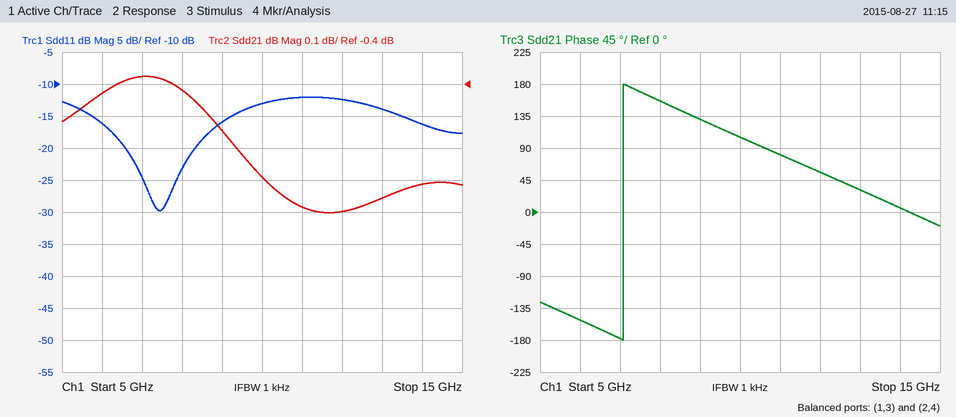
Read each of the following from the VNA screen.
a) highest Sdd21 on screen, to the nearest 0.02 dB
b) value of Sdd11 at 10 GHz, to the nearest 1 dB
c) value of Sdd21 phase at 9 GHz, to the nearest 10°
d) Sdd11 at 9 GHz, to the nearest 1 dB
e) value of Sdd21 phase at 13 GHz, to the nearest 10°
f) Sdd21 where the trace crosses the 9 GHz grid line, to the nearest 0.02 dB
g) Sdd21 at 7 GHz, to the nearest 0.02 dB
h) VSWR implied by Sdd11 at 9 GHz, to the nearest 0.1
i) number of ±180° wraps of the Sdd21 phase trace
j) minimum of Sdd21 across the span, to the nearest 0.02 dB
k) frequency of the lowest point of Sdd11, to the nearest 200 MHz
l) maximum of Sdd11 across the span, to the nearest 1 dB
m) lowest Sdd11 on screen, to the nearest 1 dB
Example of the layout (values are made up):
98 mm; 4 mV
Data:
-0.38 dB; -13 dB; 130°; -16 dB; 30°; -0.54 dB; -0.38 dB; 1.4; 1; -0.80 dB; 7.4 GHz; -12 dB; -30 dB
